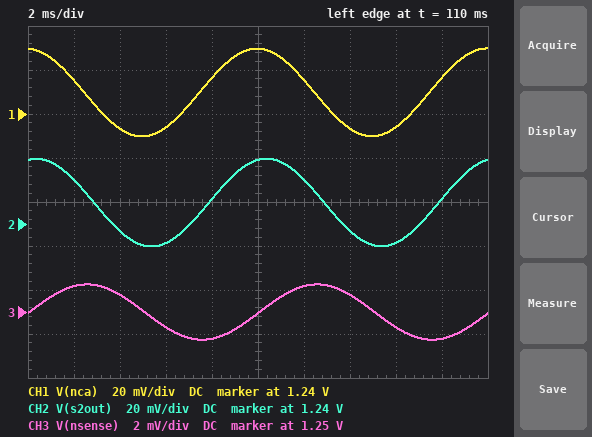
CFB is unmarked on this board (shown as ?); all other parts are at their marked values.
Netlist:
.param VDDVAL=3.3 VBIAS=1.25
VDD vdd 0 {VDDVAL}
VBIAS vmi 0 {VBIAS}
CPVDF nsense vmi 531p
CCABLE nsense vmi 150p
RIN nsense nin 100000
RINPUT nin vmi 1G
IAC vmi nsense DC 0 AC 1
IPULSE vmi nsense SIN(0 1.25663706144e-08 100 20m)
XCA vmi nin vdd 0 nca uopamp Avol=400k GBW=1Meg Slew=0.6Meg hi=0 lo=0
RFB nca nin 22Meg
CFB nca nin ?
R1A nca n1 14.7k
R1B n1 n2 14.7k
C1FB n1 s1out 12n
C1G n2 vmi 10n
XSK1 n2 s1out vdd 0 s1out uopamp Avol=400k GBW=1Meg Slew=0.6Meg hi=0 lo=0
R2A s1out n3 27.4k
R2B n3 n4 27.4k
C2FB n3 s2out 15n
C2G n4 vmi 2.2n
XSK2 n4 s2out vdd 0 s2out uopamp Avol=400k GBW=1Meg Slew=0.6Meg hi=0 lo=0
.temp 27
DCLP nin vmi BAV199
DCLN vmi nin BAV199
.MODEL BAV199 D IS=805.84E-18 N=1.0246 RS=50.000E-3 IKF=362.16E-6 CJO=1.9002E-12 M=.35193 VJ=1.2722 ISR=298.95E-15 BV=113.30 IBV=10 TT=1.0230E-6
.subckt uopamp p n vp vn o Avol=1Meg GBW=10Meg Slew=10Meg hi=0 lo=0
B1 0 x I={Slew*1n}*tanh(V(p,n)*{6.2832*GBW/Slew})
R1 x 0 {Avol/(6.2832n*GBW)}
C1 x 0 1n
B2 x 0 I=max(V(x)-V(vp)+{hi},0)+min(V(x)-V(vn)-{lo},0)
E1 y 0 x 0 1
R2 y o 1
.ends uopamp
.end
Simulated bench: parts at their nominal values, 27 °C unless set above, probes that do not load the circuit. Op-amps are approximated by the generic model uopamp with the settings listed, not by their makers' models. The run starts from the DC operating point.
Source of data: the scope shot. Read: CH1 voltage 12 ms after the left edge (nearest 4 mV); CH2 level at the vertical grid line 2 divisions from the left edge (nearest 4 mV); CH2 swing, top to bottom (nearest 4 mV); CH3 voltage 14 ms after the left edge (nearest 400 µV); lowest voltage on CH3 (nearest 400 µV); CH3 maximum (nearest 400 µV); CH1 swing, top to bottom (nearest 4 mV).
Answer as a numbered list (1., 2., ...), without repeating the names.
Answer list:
1. 1.256 V
2. 1.236 V
3. 40 mV
4. 1.2508 V
5. 1.2488 V
6. 1.2512 V
7. 40 mV
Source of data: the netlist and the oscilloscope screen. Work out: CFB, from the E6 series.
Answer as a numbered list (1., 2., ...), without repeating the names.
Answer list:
1. 1 nF
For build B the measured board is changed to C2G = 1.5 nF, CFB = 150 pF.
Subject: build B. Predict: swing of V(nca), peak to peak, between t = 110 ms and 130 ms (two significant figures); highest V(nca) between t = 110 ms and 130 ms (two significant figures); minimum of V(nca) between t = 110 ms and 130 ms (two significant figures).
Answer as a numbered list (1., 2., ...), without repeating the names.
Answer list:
1. 240 mV
2. 1.4 V
3. 1.1 V
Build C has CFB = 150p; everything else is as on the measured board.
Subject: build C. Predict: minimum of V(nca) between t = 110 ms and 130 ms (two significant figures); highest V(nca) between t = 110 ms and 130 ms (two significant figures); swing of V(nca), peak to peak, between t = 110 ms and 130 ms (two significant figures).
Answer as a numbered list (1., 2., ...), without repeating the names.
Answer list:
1. 1.1 V
2. 1.4 V
3. 240 mV
